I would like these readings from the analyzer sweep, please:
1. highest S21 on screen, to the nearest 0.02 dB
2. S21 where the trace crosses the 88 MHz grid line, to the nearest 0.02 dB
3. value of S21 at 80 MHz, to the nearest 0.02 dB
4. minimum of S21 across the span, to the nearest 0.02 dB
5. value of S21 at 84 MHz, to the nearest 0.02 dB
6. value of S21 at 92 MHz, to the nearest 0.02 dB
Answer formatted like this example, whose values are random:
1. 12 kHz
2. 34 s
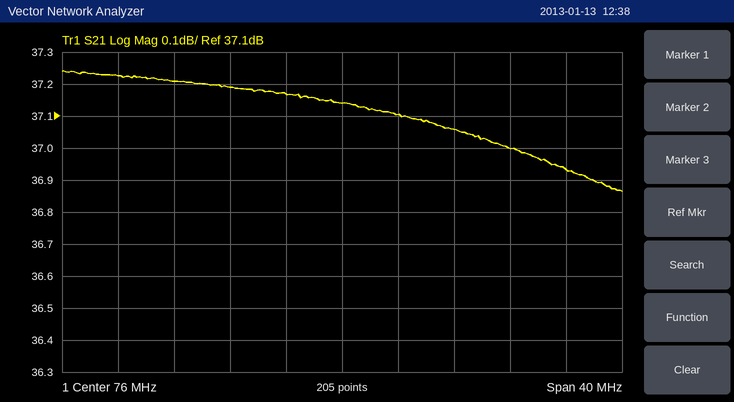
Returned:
1. 37.24 dB
2. 37.00 dB
3. 37.10 dB
4. 36.86 dB
5. 37.06 dB
6. 36.94 dB
